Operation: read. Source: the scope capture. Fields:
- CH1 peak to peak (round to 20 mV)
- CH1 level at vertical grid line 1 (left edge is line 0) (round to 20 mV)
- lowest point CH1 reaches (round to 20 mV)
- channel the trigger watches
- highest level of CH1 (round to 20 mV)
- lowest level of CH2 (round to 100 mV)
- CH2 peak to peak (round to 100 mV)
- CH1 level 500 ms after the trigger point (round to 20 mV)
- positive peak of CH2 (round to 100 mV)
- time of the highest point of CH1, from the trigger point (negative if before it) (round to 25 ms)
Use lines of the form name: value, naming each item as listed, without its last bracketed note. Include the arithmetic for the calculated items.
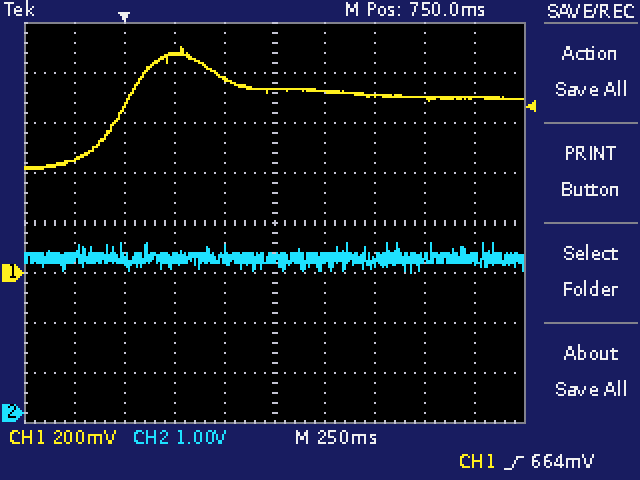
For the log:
CH1 peak to peak: 900 mV − (420 mV) = 480 mV
CH1 level at vertical grid line 1 (left edge is line 0): 460 mV
lowest point CH1 reaches: 420 mV
channel the trigger watches: CH1
highest level of CH1: 900 mV
lowest level of CH2: 2.8 V
CH2 peak to peak: 3.4 V − (2.8 V) = 600 mV
CH1 level 500 ms after the trigger point: 780 mV
positive peak of CH2: 3.4 V
time of the highest point of CH1, from the trigger point (negative if before it): +300 ms
